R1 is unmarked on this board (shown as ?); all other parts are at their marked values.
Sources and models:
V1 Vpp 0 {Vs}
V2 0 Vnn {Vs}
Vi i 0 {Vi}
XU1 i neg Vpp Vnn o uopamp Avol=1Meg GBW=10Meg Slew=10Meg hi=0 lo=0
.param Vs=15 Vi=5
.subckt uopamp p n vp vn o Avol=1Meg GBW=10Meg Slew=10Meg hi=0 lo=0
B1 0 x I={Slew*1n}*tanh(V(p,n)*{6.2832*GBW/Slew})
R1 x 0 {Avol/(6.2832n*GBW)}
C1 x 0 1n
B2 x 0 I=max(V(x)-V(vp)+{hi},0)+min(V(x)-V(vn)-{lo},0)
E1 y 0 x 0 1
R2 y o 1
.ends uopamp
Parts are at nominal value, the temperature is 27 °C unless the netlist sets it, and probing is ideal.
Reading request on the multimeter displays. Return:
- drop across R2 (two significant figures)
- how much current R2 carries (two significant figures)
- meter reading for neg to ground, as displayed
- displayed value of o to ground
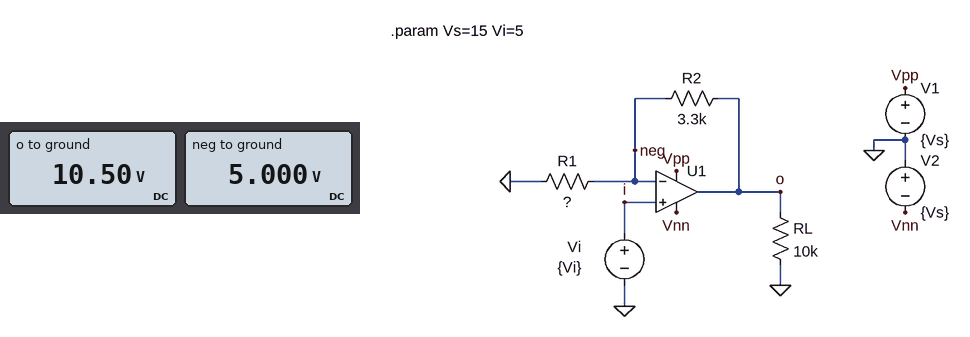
5.5 V
1.7 mA
5.000 V
10.50 V
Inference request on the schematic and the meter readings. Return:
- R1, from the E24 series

3 kΩ
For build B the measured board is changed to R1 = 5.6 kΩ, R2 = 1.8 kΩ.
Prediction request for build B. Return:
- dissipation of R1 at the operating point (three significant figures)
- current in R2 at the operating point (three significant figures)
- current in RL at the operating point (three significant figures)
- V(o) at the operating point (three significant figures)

4.46 mW
893 µA
661 µA
6.61 V
